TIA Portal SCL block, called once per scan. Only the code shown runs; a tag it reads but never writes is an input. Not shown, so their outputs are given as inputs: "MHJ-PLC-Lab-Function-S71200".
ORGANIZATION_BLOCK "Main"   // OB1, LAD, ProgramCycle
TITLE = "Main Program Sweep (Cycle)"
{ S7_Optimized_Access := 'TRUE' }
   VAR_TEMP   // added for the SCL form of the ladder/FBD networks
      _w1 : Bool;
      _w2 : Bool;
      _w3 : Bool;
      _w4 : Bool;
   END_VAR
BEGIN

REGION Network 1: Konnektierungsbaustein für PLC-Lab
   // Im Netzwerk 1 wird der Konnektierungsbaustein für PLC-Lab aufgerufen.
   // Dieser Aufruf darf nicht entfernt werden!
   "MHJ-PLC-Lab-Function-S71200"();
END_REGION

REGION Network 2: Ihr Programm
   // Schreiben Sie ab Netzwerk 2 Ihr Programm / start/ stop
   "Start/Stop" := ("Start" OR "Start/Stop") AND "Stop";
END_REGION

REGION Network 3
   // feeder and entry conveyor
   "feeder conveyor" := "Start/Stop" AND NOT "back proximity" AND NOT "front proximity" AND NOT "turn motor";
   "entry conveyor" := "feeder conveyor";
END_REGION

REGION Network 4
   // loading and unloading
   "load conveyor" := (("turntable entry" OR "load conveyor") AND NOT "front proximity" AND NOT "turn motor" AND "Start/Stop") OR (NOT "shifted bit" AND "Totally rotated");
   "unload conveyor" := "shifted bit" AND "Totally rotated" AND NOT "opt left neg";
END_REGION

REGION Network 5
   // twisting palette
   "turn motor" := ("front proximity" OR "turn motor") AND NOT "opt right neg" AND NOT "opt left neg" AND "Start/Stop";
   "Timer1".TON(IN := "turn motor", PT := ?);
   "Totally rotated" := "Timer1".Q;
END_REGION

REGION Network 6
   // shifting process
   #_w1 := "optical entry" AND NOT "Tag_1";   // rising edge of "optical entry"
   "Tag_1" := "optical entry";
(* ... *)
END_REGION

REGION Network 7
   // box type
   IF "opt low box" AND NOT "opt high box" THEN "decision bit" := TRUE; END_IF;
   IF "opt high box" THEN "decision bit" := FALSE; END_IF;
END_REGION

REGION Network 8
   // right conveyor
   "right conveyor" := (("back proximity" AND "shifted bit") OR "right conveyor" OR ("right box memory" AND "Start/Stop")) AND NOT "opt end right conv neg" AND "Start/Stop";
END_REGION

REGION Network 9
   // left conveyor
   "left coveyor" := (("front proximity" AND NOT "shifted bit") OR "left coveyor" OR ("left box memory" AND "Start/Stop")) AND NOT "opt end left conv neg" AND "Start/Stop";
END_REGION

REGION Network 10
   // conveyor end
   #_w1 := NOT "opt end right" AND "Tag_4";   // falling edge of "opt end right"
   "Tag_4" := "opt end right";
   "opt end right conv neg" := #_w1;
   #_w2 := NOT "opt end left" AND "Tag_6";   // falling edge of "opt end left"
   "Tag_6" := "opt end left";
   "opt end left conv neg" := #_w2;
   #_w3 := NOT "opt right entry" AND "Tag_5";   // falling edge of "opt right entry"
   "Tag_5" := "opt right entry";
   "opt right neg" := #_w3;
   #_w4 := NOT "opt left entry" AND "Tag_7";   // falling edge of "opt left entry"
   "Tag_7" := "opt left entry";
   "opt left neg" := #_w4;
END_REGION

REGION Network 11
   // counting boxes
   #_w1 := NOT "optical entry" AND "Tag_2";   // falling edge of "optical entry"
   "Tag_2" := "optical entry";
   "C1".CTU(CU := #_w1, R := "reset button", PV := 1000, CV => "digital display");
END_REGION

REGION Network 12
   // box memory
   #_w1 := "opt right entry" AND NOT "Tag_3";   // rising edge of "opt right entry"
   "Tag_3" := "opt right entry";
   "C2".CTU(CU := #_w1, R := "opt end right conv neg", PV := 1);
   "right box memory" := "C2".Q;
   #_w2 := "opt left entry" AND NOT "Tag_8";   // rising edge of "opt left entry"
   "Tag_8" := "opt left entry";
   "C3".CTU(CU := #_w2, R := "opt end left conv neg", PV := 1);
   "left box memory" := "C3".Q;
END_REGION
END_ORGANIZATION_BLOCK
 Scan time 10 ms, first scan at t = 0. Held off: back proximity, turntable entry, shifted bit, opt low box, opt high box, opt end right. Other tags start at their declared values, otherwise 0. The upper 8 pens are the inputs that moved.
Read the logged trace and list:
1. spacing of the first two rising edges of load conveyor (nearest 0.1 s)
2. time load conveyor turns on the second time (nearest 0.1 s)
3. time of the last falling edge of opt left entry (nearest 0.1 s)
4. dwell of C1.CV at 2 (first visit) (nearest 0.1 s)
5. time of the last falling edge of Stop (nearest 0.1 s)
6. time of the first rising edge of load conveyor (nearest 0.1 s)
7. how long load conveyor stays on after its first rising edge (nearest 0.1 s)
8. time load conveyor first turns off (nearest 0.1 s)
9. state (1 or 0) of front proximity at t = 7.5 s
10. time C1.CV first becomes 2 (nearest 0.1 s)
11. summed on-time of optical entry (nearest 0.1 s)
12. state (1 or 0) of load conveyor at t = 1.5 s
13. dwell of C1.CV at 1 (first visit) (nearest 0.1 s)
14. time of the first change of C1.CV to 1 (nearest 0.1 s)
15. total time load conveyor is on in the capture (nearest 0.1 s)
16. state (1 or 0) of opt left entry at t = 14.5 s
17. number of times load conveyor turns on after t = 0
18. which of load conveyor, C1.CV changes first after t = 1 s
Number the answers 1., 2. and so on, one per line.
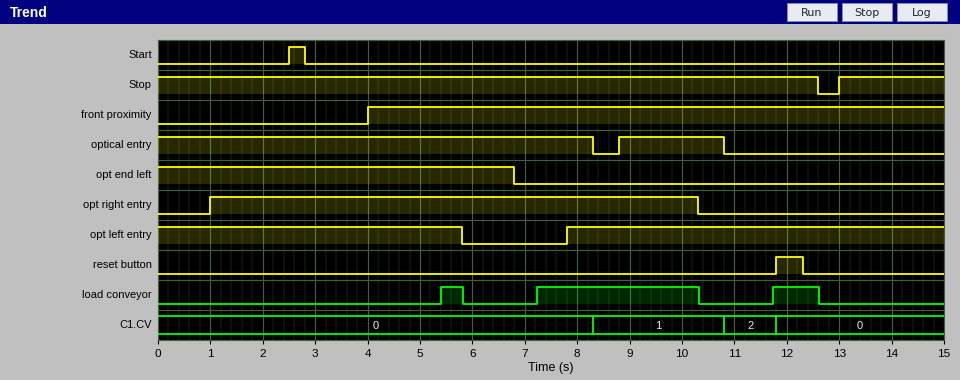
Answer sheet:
1. 1.8 s
2. 7.2 s
3. 5.8 s
4. 1.0 s
5. 12.6 s
6. 5.4 s
7. 0.4 s
8. 5.8 s
9. 1
10. 10.8 s
11. 10.3 s
12. 0
13. 2.5 s
14. 8.3 s
15. 4.4 s
16. 1
17. 3
18. load conveyor
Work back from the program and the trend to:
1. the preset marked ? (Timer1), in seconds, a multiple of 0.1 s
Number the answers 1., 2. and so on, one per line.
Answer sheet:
1. 1.4 s
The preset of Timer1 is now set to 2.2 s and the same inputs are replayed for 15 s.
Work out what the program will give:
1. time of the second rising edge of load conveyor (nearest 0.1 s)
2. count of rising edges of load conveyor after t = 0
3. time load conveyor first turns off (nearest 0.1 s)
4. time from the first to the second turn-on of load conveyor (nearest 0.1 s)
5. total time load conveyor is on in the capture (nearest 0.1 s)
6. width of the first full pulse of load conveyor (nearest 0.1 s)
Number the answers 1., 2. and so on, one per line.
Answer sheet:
1. 12.5 s
2. 2
3. 10.3 s
4. 4.5 s
5. 2.4 s
6. 2.3 s
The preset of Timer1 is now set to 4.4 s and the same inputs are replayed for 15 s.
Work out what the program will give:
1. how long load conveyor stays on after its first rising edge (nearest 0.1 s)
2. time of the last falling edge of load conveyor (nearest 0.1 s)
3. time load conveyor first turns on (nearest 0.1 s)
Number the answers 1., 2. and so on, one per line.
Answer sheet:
1. 0.1 s
2. 10.3 s
3. 10.2 s
